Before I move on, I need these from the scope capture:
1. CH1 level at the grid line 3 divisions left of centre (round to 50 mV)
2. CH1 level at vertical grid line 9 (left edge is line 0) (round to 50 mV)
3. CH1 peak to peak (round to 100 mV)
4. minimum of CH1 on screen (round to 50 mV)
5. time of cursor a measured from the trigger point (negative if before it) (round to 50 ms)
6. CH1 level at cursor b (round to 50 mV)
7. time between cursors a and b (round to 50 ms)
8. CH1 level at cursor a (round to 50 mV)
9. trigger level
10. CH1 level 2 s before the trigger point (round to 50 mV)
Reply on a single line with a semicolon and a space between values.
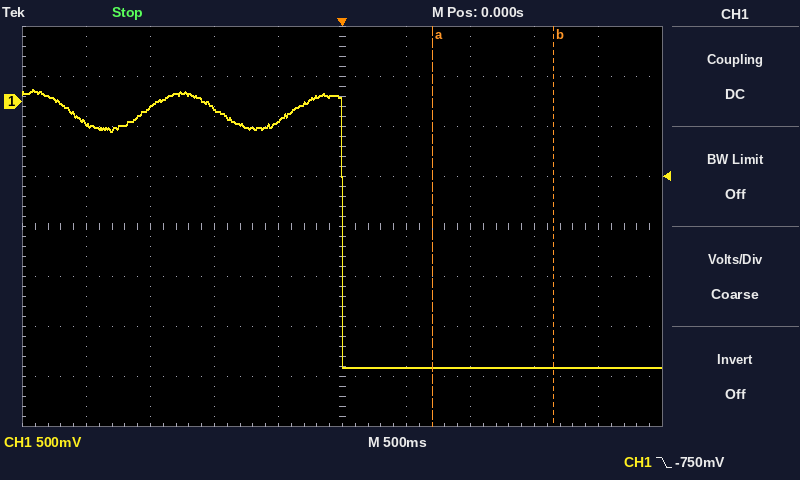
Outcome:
-50 mV; -2.65 V; 2.80 V; -2.65 V; +700 ms; -2.65 V; 950 ms; -2.65 V; -750 mV; -200 mV
